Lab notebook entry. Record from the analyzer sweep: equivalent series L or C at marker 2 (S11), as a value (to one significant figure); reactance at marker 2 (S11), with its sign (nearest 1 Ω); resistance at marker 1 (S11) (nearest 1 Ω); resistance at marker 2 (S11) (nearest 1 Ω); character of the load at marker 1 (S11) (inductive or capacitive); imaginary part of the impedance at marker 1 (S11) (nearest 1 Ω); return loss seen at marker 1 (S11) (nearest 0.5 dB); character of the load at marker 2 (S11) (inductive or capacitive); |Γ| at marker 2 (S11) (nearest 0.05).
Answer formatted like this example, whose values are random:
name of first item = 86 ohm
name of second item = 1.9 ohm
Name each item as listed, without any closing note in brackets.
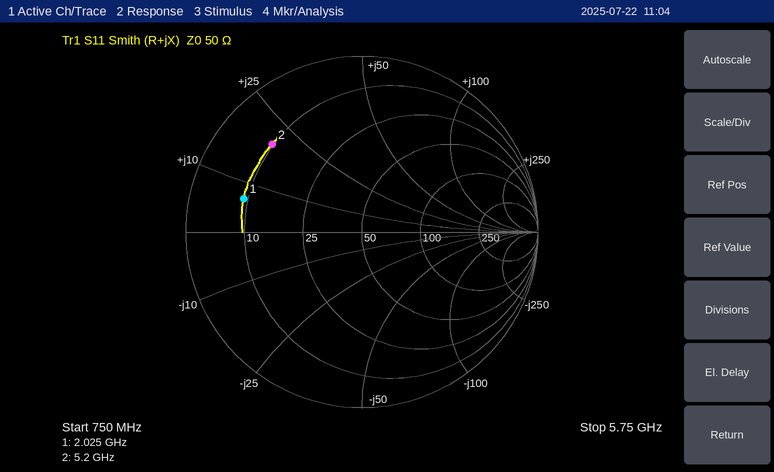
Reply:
equivalent series L or C at marker 2 (S11), as a value = 600 pH
reactance at marker 2 (S11), with its sign = +20 Ω
resistance at marker 1 (S11) = 9 Ω
resistance at marker 2 (S11) = 10 Ω
character of the load at marker 1 (S11) = inductive
imaginary part of the impedance at marker 1 (S11) = +7 Ω
return loss seen at marker 1 (S11) = 3.0 dB
character of the load at marker 2 (S11) = inductive
|Γ| at marker 2 (S11) = 0.70
